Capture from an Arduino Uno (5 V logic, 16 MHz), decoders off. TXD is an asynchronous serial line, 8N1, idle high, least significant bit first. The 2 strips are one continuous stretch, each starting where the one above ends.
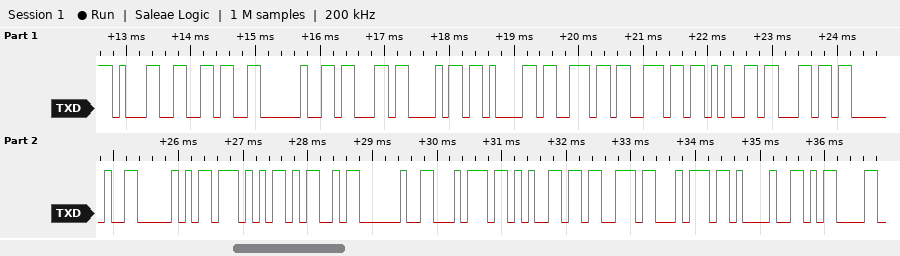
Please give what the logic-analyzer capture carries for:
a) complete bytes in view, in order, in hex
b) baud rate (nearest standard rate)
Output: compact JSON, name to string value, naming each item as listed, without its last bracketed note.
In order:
{"complete bytes in view, in order, in hex": "31 36 20 63 68 61 6E 6E 65 6C 20 50 57 4D 20 74 65 73 74 21 0D", "baud rate": "9600 baud"}
